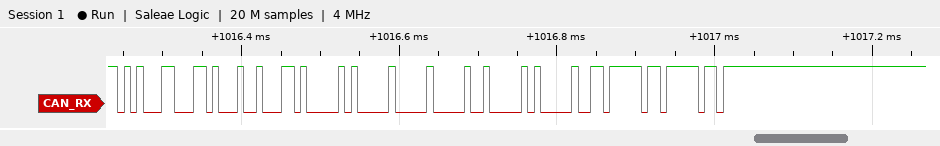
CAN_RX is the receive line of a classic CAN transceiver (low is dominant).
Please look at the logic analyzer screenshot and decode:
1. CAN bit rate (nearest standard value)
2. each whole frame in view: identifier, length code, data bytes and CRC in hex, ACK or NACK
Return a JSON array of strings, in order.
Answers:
["125 kbit/s", "ID 14611234, DLC 4, data 00 01 02 03, CRC 3FBF, ACK"]
